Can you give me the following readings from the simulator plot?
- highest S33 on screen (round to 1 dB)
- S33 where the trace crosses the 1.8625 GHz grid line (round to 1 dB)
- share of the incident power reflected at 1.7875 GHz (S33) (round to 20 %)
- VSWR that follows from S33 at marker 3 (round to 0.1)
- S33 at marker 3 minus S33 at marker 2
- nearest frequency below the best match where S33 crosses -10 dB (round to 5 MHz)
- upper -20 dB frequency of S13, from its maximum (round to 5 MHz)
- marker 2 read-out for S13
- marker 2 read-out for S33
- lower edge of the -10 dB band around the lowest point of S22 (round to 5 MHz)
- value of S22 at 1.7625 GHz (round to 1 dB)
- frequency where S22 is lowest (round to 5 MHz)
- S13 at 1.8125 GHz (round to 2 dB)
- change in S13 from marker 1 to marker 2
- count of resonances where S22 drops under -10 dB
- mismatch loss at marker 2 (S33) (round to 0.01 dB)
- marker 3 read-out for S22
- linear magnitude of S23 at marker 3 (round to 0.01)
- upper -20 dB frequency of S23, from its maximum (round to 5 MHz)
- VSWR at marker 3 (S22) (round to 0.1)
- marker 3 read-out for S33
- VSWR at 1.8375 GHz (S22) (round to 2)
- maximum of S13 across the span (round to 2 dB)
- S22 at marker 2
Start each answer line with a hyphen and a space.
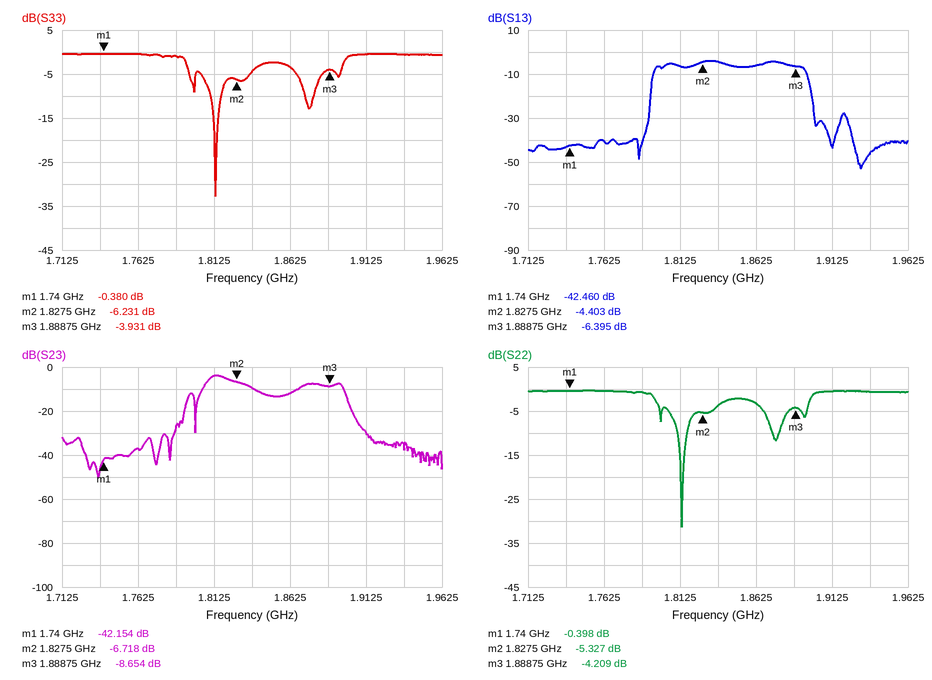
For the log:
- 0 dB
- -3 dB
- 80 %
- 4.5
- 2.300 dB
- 1.810 GHz
- 1.900 GHz
- -4.403 dB
- -6.231 dB
- 1.810 GHz
- 0 dB
- 1.815 GHz
- -6 dB
- 38.057 dB
- 2
- 1.18 dB
- -4.209 dB
- 0.37
- 1.905 GHz
- 4.2
- -3.931 dB
- 4
- -4 dB
- -5.327 dB
